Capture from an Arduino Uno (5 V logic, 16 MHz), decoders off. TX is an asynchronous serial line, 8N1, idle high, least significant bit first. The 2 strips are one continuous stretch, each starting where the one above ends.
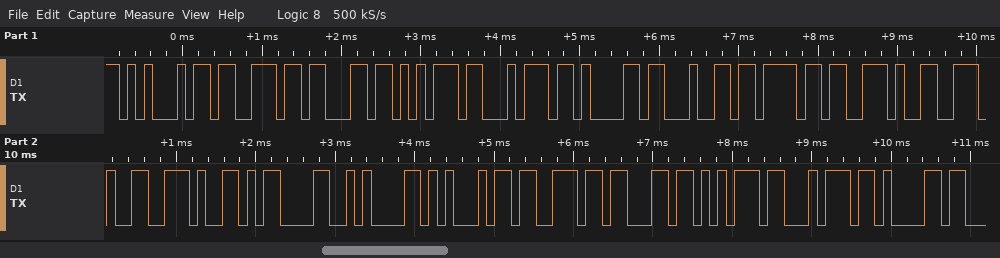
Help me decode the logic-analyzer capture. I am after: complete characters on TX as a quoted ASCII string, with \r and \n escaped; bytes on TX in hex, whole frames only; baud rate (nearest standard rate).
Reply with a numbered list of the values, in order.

1. "Escutado...\r\nEscuta"
2. 45 73 63 75 74 61 64 6F 2E 2E 2E 0D 0A 45 73 63 75 74 61
3. 9600 baud
